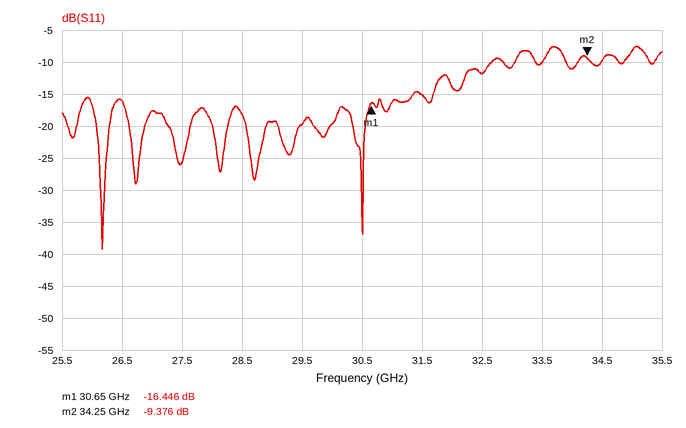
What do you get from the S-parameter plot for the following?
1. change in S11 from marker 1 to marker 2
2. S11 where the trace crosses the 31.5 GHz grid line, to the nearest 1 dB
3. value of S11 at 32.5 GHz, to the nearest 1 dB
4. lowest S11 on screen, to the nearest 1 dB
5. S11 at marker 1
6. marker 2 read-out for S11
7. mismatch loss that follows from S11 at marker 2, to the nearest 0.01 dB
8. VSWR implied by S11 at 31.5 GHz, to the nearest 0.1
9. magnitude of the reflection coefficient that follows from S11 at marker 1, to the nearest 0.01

7.070 dB
-15 dB
-12 dB
-39 dB
-16.446 dB
-9.376 dB
0.53 dB
1.4
0.15
